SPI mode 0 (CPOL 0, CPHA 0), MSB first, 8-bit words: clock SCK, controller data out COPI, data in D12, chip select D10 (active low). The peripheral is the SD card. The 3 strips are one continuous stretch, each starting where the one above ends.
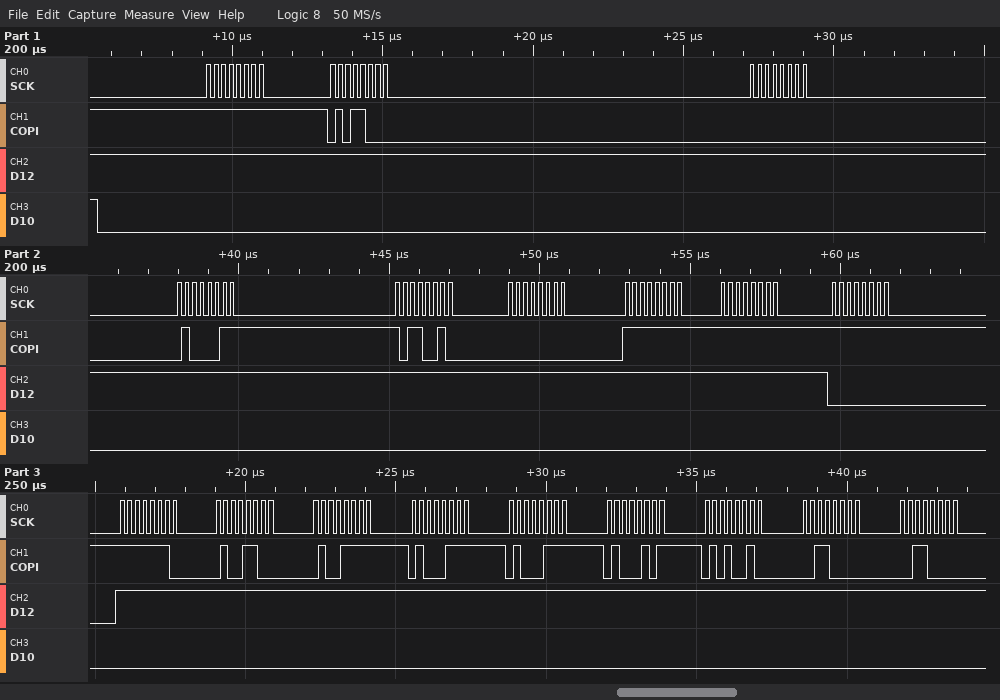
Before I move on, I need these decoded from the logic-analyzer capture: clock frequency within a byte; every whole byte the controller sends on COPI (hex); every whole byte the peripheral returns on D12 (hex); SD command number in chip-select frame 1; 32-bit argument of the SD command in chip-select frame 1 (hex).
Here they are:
4 MHz
0xFF 0x58 0x00 0x43 0xB2 0x00 0xFF 0xFF 0xFF 0xFE 0x4C 0x4F 0x47 0x47 0x45 0x52 0x30 0x30
0xFF 0xFF 0xFF 0xFF 0xFF 0xFF 0xFF 0xFF 0x00 0xFF 0xFF 0xFF 0xFF 0xFF 0xFF 0xFF 0xFF 0xFF
CMD24
0x0043B200
